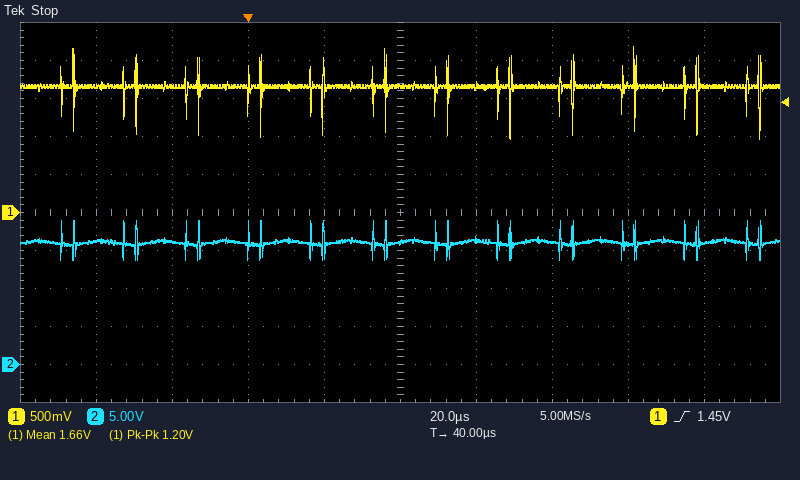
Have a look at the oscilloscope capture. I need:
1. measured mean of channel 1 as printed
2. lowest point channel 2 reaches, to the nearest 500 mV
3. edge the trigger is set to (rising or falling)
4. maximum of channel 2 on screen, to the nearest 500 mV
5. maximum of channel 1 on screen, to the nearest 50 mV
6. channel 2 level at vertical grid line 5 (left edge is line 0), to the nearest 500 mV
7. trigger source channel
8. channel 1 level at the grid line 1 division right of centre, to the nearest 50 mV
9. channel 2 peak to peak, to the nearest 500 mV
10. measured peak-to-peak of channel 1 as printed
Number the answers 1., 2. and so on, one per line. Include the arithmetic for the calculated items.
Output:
1. 1.66 V
2. 14.0 V
3. rising
4. 19.0 V
5. 2.20 V
6. 16.0 V
7. channel 1
8. 1.65 V
9. 19.0 V − (14.0 V) = 5.0 V
10. 1.20 V
